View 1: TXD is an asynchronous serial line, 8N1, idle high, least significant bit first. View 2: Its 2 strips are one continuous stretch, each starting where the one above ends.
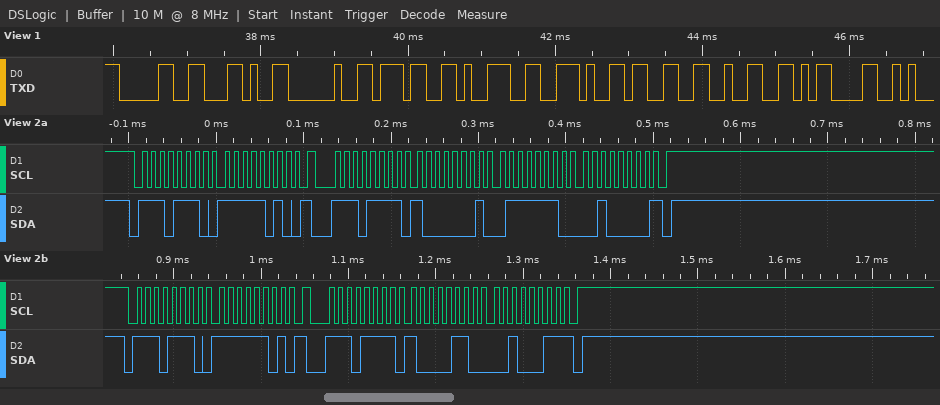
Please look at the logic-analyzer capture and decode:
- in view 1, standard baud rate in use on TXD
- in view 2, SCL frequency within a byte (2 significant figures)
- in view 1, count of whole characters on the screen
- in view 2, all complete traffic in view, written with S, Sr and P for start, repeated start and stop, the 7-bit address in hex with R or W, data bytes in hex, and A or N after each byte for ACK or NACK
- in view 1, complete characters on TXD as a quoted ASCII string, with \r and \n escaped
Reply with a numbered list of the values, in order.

1. 9600 baud
2. 100 kHz
3. 9
4. S 77W A FA A Sr 77R A 81 A 7E A 20 N P S 77W A FD A Sr 77R A 86 A 23 N P
5. "0, 79.32\r"
